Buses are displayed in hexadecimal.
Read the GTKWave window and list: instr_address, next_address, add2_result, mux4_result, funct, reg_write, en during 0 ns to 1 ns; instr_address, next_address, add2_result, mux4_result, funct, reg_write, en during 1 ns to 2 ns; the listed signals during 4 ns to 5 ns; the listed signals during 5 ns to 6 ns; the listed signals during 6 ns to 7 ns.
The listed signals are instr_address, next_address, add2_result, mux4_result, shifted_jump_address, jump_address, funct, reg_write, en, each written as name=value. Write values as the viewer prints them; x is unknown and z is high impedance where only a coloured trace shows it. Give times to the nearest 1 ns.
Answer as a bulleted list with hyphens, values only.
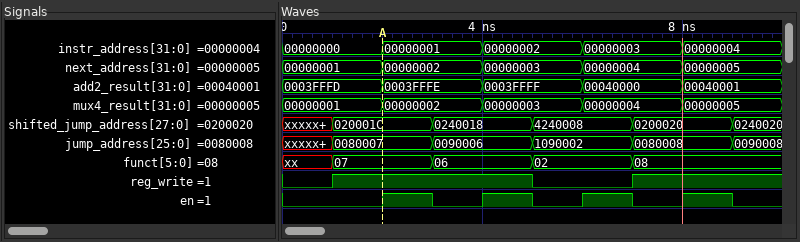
- instr_address=00000000, next_address=00000001, add2_result=0003FFFD, mux4_result=00000001, funct=xx, reg_write=0, en=0
- instr_address=00000000, next_address=00000001, add2_result=0003FFFD, mux4_result=00000001, funct=07, reg_write=1, en=0
- instr_address=00000002, next_address=00000003, add2_result=0003FFFF, mux4_result=00000003, shifted_jump_address=0240018, jump_address=0090006, funct=06, reg_write=1, en=1
- instr_address=00000002, next_address=00000003, add2_result=0003FFFF, mux4_result=00000003, shifted_jump_address=4240008, jump_address=1090002, funct=02, reg_write=0, en=0
- instr_address=00000003, next_address=00000004, add2_result=00040000, mux4_result=00000004, shifted_jump_address=4240008, jump_address=1090002, funct=02, reg_write=0, en=1
